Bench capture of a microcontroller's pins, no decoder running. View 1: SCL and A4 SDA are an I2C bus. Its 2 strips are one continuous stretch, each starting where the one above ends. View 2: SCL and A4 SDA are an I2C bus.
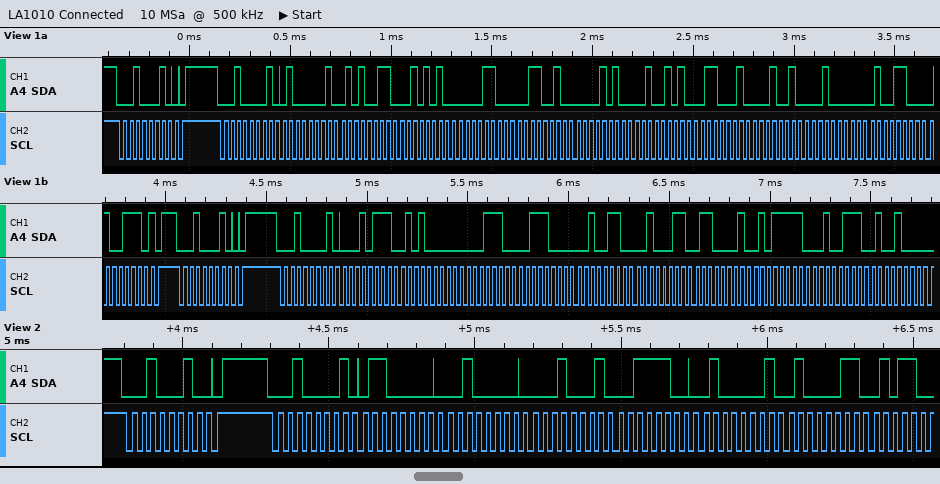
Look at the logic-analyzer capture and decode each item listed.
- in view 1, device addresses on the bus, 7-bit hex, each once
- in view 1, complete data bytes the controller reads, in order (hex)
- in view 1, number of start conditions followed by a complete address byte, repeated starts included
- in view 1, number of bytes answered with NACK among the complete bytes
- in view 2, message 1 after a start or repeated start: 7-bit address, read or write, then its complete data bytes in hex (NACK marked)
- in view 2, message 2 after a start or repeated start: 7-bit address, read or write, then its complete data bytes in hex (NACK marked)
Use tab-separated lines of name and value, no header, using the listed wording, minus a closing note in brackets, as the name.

in view 1, device addresses on the bus, 7-bit hex, each once	0x11 0x10
in view 1, complete data bytes the controller reads, in order	41 53 2A 0C 32 0A 25 31 12 20 4C 4E 17 50 0E 38 26 23 61 5F 27 48
in view 1, number of start conditions followed by a complete address byte, repeated starts included	4
in view 1, number of bytes answered with NACK among the complete bytes	1
in view 2, message 1 after a start or repeated start: 7-bit address, read or write, then its complete data bytes in hex	0x11 write
in view 2, message 2 after a start or repeated start: 7-bit address, read or write, then its complete data bytes in hex	0x10 read: 60 20 11 3C 41 43
